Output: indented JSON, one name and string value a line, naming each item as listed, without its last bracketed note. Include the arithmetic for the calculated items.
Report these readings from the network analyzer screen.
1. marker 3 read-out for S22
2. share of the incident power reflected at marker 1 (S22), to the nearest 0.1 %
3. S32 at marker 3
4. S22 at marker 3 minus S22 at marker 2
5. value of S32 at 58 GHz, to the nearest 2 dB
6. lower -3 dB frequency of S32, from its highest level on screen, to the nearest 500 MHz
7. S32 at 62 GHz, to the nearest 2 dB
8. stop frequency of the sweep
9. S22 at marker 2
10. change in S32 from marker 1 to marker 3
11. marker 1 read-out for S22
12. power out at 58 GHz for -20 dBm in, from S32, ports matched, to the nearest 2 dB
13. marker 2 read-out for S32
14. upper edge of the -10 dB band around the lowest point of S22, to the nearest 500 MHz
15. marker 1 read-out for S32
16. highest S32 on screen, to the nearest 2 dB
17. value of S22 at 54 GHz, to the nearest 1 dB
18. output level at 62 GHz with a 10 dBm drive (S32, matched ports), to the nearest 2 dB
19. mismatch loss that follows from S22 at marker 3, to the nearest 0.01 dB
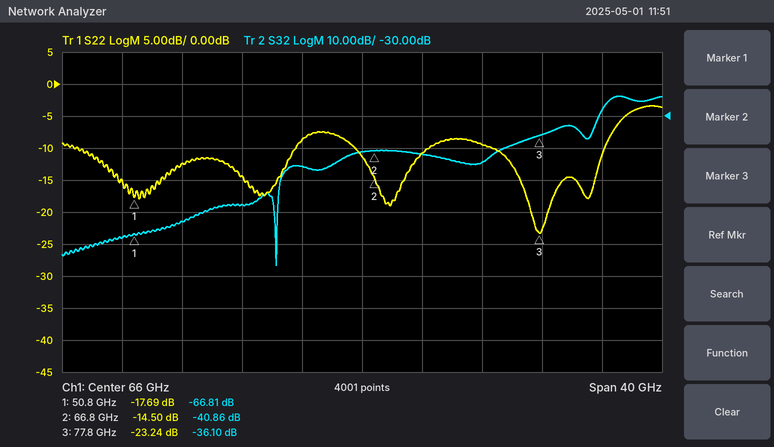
{
  "marker 3 read-out for S22": "-23.24 dB",
  "share of the incident power reflected at marker 1 (S22), to the nearest 0.1 %": "10^(-17.69/10) ≈ 1.7 %",
  "S32 at marker 3": "-36.10 dB",
  "S22 at marker 3 minus S22 at marker 2": "-23.24 − (-14.5) = -8.74 dB",
  "value of S32 at 58 GHz, to the nearest 2 dB": "-58 dB",
  "lower -3 dB frequency of S32, from its highest level on screen, to the nearest 500 MHz": "82.0 GHz",
  "S32 at 62 GHz, to the nearest 2 dB": "-46 dB",
  "stop frequency of the sweep": "86 GHz",
  "S22 at marker 2": "-14.50 dB",
  "change in S32 from marker 1 to marker 3": "-36.1 − (-66.81) = 30.71 dB",
  "marker 1 read-out for S22": "-17.69 dB",
  "power out at 58 GHz for -20 dBm in, from S32, ports matched, to the nearest 2 dB": "-20 dBm + (-58 dB) = -78 dBm",
  "marker 2 read-out for S32": "-40.86 dB",
  "upper edge of the -10 dB band around the lowest point of S22, to the nearest 500 MHz": "82.0 GHz",
  "marker 1 read-out for S32": "-66.81 dB",
  "highest S32 on screen, to the nearest 2 dB": "-24 dB",
  "value of S22 at 54 GHz, to the nearest 1 dB": "-12 dB",
  "output level at 62 GHz with a 10 dBm drive (S32, matched ports), to the nearest 2 dB": "10 dBm + (-46 dB) = -36 dBm",
  "mismatch loss that follows from S22 at marker 3, to the nearest 0.01 dB": "−10 log10(1 − 10^(-23.24/10)) ≈ 0.02 dB"
}
